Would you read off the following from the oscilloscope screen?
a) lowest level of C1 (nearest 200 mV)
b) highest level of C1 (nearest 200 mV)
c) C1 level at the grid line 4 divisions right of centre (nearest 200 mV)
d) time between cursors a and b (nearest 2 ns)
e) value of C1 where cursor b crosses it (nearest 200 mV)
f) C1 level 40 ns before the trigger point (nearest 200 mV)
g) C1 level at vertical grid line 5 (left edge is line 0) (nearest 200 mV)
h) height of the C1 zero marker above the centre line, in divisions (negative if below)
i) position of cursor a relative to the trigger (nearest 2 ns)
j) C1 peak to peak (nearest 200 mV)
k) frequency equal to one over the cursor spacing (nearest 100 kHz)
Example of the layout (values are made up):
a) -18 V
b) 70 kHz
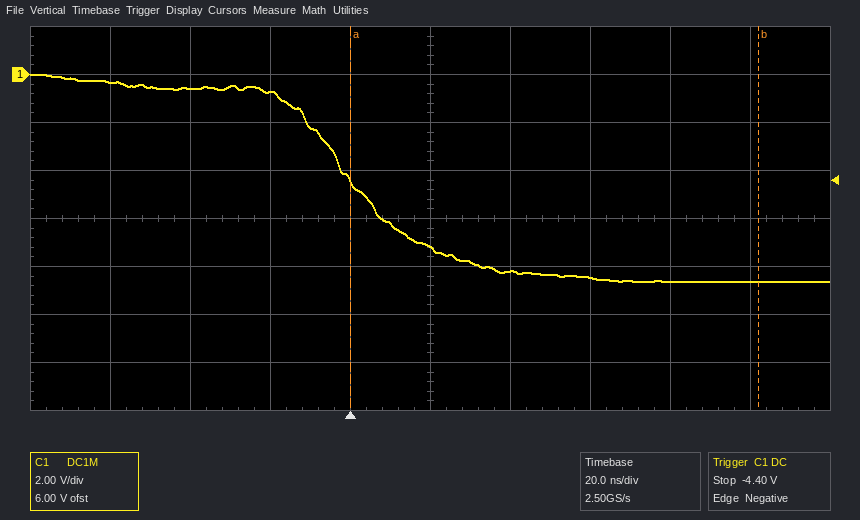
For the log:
a) -8.6 V
b) 0.0 V
c) -8.6 V
d) 102 ns
e) -8.6 V
f) -600 mV
g) -7.2 V
h) +3.0 div
i) 0 ns
j) 8.6 V
k) 9.8 MHz
